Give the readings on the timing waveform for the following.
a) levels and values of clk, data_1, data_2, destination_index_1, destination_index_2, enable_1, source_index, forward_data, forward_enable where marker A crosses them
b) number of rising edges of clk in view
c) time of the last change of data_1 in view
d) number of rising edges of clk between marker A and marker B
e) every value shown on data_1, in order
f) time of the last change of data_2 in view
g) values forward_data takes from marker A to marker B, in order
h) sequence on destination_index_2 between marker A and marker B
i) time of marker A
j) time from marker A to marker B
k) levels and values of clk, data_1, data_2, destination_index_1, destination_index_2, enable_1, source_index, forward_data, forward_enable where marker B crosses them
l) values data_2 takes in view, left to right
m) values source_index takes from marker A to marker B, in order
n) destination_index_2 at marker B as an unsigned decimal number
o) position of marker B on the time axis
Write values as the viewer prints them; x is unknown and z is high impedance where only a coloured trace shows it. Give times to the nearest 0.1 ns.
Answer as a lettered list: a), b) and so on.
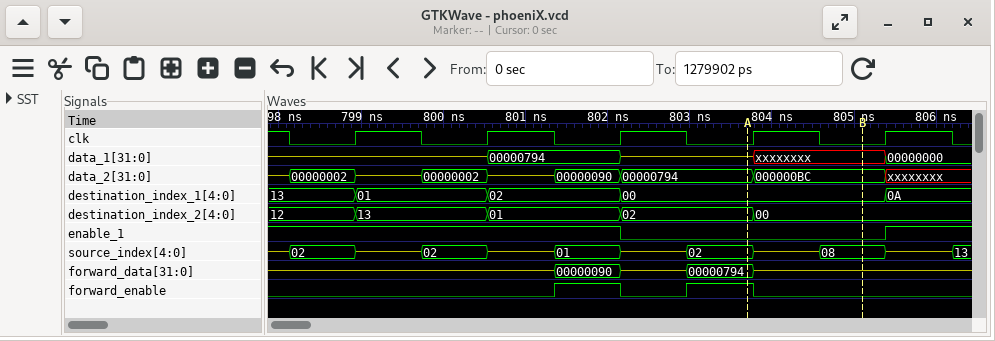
a) clk=0, data_1=z, data_2=00000794, destination_index_1=00, destination_index_2=02, enable_1=0, source_index=02, forward_data=00000794, forward_enable=1
b) 5
c) 805.4 ns
d) 1
e) z, 00000794, z, xxxxxxxx, 00000000
f) 805.4 ns
g) 00000794, z
h) 02, 00
i) 803.7 ns
j) 1.4 ns
k) clk=0, data_1=xxxxxxxx, data_2=000000BC, destination_index_1=00, destination_index_2=00, enable_1=0, source_index=08, forward_data=z, forward_enable=0
l) z, 00000002, z, 00000002, z, 00000090, 00000794, 000000BC, xxxxxxxx
m) 02, z, 08
n) 0
o) 805.1 ns
